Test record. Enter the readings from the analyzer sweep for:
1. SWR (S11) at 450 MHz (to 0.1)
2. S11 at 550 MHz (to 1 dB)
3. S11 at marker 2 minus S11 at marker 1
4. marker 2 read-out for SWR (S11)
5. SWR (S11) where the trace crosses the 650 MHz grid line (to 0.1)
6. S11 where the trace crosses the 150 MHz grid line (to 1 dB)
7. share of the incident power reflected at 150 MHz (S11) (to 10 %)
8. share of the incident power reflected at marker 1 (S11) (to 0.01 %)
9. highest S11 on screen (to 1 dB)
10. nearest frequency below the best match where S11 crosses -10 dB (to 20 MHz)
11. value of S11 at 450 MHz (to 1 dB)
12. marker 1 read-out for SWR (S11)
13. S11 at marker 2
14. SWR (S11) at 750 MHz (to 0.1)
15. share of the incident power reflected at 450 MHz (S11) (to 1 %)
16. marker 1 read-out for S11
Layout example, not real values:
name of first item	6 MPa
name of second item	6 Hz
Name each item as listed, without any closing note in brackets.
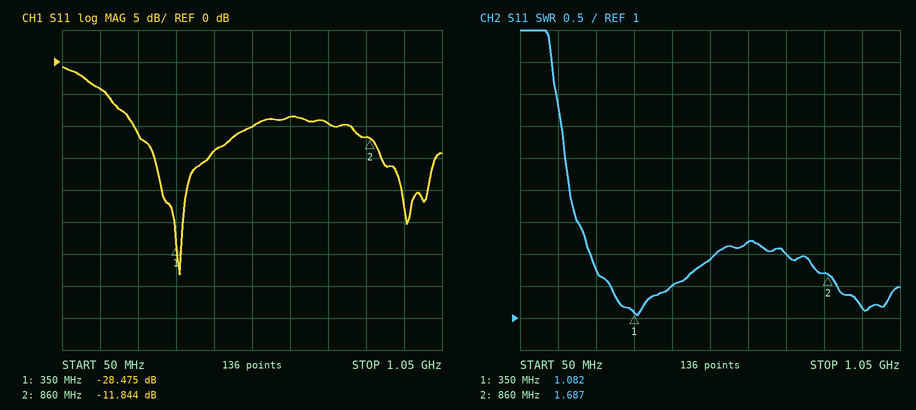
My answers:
SWR (S11) at 450 MHz	1.5
S11 at 550 MHz	-10 dB
S11 at marker 2 minus S11 at marker 1	16.631 dB
marker 2 read-out for SWR	1.687
SWR (S11) where the trace crosses the 650 MHz grid line	2.2
S11 where the trace crosses the 150 MHz grid line	-4 dB
share of the incident power reflected at 150 MHz (S11)	40 %
share of the incident power reflected at marker 1 (S11)	0.14 %
highest S11 on screen	-1 dB
nearest frequency below the best match where S11 crosses -10 dB	240 MHz
value of S11 at 450 MHz	-14 dB
marker 1 read-out for SWR	1.082
S11 at marker 2	-11.844 dB
SWR (S11) at 750 MHz	2.0
share of the incident power reflected at 450 MHz (S11)	4 %
marker 1 read-out for S11	-28.475 dB
